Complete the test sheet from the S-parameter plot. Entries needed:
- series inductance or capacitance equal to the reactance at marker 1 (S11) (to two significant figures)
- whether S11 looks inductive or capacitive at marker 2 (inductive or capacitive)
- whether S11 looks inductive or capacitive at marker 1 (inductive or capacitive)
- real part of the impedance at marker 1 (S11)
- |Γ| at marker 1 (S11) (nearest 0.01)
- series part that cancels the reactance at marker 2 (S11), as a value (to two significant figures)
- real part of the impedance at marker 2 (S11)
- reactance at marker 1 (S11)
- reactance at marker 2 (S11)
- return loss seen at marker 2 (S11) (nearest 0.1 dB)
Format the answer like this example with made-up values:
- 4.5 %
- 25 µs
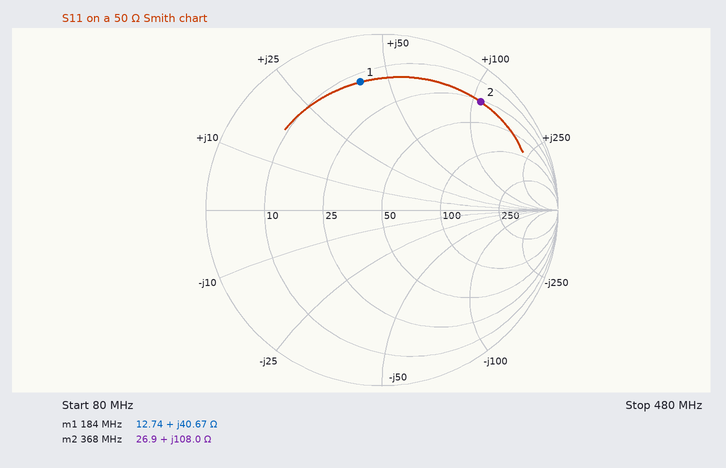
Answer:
- 35 nH
- inductive
- inductive
- 12.74 Ω
- 0.74
- 4.0 pF
- 26.9 Ω
- +40.67 Ω
- +108.0 Ω
- 1.6 dB
